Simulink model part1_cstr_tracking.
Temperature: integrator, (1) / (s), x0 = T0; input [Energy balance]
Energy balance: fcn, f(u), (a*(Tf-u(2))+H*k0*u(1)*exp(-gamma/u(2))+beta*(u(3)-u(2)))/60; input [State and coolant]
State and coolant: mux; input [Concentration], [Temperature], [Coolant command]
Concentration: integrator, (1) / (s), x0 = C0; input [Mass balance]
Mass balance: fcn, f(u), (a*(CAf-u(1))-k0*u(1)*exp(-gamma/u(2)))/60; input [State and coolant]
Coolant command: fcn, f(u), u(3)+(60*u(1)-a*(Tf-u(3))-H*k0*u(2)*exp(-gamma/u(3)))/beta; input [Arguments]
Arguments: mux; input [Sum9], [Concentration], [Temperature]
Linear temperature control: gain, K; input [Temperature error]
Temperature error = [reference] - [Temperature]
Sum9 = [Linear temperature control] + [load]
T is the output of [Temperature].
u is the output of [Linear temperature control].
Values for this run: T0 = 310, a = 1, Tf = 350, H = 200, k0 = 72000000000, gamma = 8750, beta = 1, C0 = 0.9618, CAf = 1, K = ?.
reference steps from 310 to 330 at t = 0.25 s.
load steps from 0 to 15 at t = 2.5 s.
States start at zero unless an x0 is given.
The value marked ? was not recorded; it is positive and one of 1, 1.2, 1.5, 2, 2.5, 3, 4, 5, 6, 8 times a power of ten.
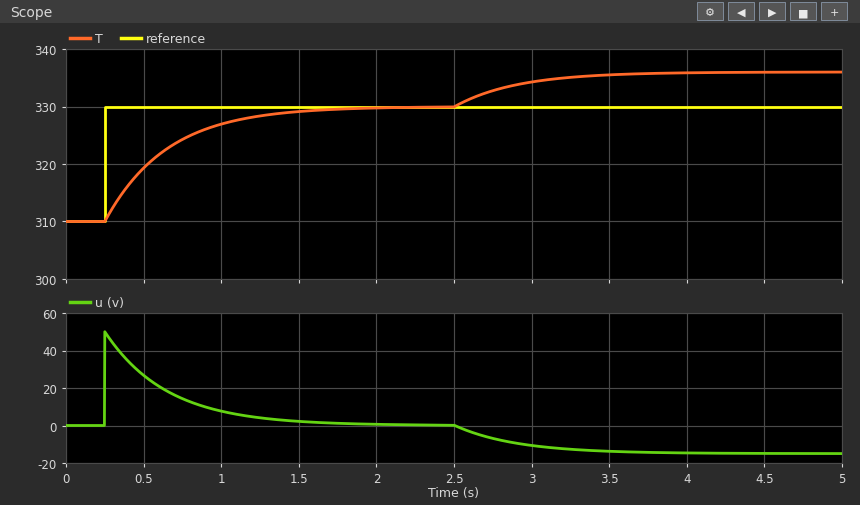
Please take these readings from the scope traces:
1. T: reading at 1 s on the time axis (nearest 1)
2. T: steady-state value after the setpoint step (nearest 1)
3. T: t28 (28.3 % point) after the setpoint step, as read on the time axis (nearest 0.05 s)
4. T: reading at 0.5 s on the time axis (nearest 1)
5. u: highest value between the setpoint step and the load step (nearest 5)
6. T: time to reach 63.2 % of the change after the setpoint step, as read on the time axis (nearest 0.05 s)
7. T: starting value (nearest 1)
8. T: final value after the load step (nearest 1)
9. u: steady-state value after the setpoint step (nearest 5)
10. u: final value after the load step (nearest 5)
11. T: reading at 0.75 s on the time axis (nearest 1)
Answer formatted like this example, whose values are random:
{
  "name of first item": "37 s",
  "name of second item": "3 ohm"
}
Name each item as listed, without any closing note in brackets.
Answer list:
{
  "T: reading at 1 s on the time axis": "327",
  "T: steady-state value after the setpoint step": "330",
  "T: t28 (28.3 % point) after the setpoint step, as read on the time axis": "0.40 s",
  "T: reading at 0.5 s on the time axis": "319",
  "u: highest value between the setpoint step and the load step": "50",
  "T: time to reach 63.2 % of the change after the setpoint step, as read on the time axis": "0.65 s",
  "T: starting value": "310",
  "T: final value after the load step": "336",
  "u: steady-state value after the setpoint step": "0",
  "u: final value after the load step": "-15",
  "T: reading at 0.75 s on the time axis": "324"
}
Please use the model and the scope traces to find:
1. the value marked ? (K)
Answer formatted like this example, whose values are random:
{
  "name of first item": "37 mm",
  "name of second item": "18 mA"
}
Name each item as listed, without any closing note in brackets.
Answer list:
{
  "the value marked ?": "2.5"
}
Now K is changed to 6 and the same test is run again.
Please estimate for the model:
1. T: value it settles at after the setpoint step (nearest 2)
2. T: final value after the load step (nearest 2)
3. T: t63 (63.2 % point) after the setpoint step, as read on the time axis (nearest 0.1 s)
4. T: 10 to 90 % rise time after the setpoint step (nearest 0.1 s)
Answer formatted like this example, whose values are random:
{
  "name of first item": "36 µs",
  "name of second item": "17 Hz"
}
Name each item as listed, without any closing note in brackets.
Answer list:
{
  "T: value it settles at after the setpoint step": "330",
  "T: final value after the load step": "332",
  "T: t63 (63.2 % point) after the setpoint step, as read on the time axis": "0.4 s",
  "T: 10 to 90 % rise time after the setpoint step": "0.4 s"
}
